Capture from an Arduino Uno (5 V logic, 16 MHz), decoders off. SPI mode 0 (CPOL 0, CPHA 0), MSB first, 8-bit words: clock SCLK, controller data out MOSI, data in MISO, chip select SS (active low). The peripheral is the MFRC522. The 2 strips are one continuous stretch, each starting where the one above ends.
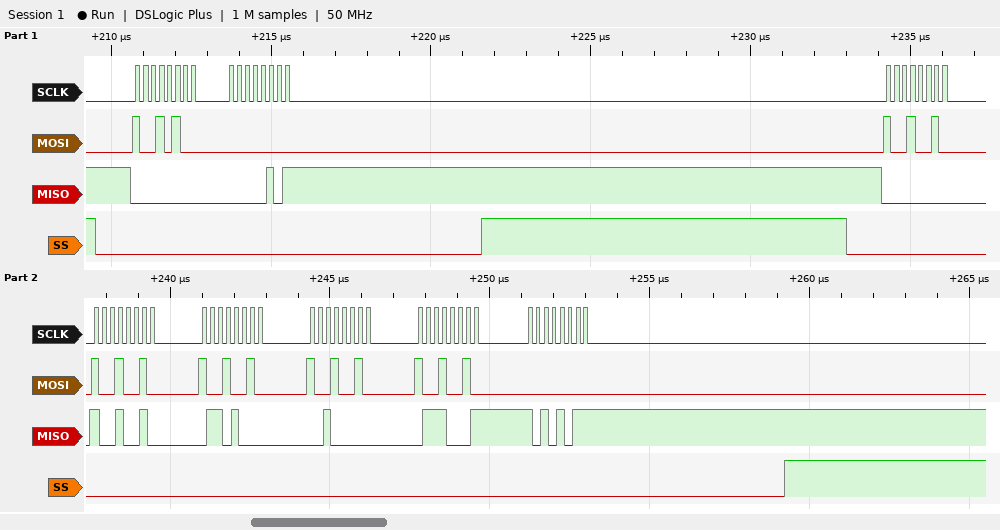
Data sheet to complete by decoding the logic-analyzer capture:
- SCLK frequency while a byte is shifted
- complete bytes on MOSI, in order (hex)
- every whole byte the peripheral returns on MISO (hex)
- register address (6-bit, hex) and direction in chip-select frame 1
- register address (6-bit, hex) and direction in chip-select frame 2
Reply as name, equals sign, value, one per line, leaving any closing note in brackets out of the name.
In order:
SCLK frequency while a byte is shifted = 4 MHz
complete bytes on MOSI, in order = 94 00 92 92 92 92 92 00
every whole byte the peripheral returns on MISO = 00 05 00 92 68 20 71 AB
register address (6-bit, hex) and direction in chip-select frame 1 = 0x0A read
register address (6-bit, hex) and direction in chip-select frame 2 = 0x09 read
